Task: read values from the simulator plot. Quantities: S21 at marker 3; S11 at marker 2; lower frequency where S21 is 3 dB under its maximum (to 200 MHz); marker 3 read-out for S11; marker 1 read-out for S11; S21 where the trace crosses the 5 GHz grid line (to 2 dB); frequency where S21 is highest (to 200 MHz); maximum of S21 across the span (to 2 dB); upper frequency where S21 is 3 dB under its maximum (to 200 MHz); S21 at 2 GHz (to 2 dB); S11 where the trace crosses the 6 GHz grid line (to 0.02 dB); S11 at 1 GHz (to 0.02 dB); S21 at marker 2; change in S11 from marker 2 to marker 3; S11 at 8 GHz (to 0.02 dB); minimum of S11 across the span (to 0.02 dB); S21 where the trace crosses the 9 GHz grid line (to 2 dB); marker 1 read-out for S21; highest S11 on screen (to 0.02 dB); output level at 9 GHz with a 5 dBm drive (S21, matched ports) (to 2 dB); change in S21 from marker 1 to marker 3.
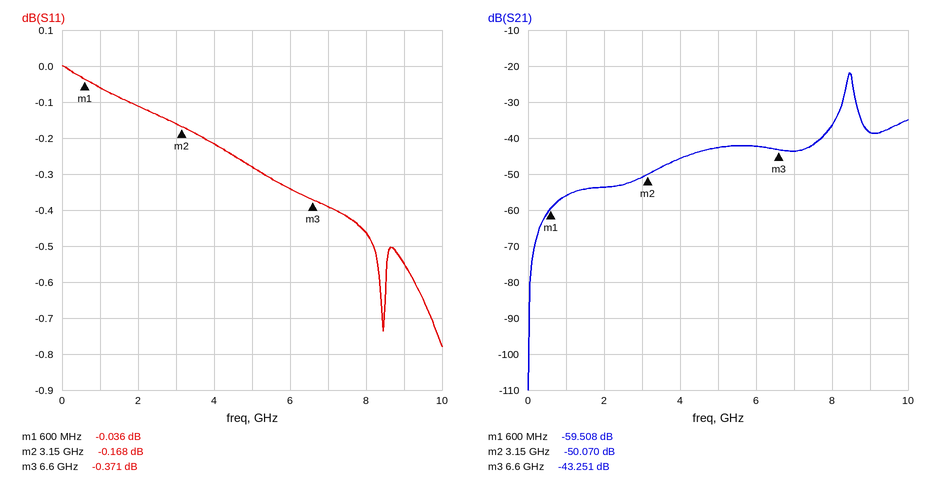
-43.251 dB
-0.168 dB
8.4 GHz
-0.371 dB
-0.036 dB
-42 dB
8.4 GHz
-22 dB
8.6 GHz
-54 dB
-0.34 dB
-0.06 dB
-50.070 dB
-0.203 dB
-0.46 dB
-0.78 dB
-38 dB
-59.508 dB
0.00 dB
-34 dBm
16.257 dB
